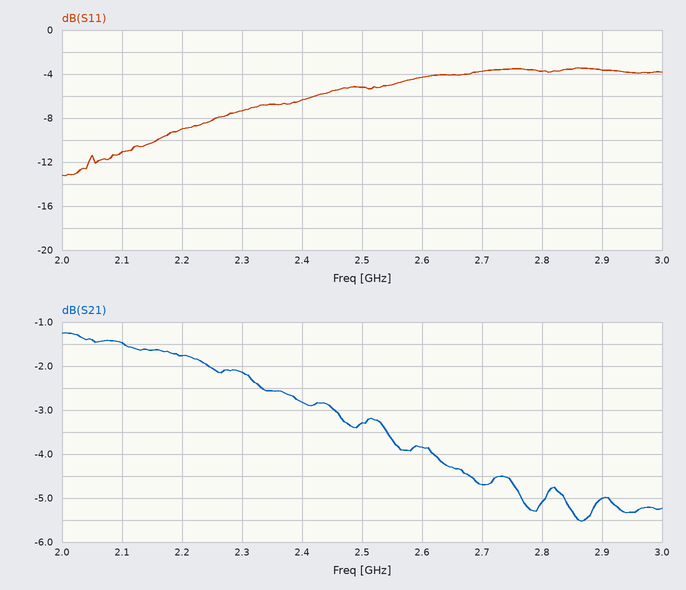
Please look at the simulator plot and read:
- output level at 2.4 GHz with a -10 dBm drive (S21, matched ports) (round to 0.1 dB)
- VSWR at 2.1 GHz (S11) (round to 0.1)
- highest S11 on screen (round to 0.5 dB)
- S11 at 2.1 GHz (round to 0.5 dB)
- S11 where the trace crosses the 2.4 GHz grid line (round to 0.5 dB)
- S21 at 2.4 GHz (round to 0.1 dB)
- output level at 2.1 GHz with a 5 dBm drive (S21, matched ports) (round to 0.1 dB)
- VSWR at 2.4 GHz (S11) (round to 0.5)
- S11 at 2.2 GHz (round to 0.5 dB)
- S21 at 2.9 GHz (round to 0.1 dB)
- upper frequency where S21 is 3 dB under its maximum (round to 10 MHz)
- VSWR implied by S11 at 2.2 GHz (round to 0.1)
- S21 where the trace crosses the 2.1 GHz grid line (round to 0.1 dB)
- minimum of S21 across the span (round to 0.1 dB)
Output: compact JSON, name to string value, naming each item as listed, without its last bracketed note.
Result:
{"output level at 2.4 GHz with a -10 dBm drive (S21, matched ports)": "-12.8 dBm", "VSWR at 2.1 GHz (S11)": "1.8", "highest S11 on screen": "-3.5 dB", "S11 at 2.1 GHz": "-11.0 dB", "S11 where the trace crosses the 2.4 GHz grid line": "-6.5 dB", "S21 at 2.4 GHz": "-2.8 dB", "output level at 2.1 GHz with a 5 dBm drive (S21, matched ports)": "3.5 dBm", "VSWR at 2.4 GHz (S11)": "3.0", "S11 at 2.2 GHz": "-9.0 dB", "S21 at 2.9 GHz": "-5.0 dB", "upper frequency where S21 is 3 dB under its maximum": "2.64 GHz", "VSWR implied by S11 at 2.2 GHz": "2.1", "S21 where the trace crosses the 2.1 GHz grid line": "-1.5 dB", "minimum of S21 across the span": "-5.5 dB"}
